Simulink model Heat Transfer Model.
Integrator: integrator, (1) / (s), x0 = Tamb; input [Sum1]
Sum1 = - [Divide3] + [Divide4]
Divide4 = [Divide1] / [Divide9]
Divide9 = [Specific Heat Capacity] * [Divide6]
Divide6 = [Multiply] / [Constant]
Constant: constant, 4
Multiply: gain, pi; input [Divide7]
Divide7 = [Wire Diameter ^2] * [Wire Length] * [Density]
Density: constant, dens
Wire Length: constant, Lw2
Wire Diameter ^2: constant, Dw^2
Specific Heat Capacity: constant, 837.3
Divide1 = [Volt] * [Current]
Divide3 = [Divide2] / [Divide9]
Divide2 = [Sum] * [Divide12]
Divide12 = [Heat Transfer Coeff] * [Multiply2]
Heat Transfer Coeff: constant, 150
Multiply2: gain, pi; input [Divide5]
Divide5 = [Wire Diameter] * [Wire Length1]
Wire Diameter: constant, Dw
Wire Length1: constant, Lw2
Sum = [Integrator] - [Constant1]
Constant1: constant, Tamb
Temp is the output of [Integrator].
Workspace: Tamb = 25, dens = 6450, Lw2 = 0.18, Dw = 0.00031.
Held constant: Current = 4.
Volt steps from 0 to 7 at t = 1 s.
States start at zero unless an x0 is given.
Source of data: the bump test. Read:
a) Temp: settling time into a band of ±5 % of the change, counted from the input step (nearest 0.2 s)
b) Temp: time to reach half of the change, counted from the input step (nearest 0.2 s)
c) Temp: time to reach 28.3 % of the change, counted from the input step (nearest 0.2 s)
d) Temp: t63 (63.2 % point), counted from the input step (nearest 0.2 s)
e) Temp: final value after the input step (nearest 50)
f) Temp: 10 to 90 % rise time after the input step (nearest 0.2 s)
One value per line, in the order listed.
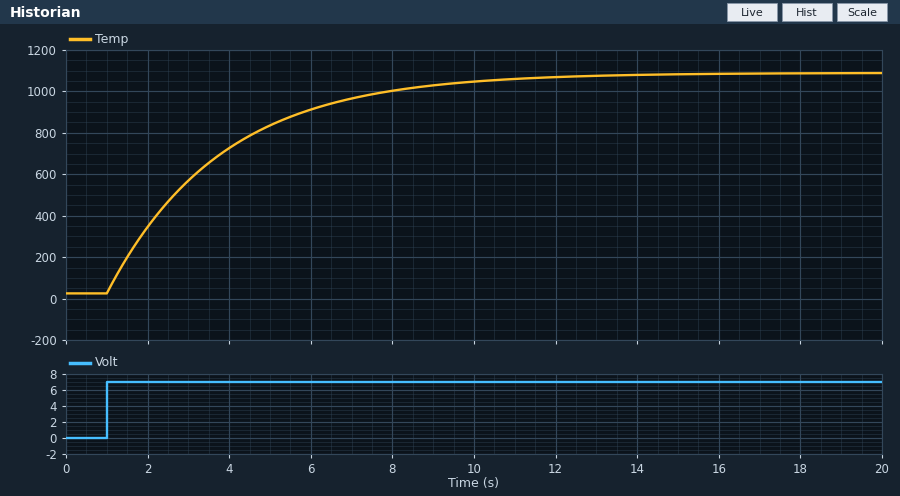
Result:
8.4 s
2.0 s
1.0 s
2.8 s
1100
6.2 s
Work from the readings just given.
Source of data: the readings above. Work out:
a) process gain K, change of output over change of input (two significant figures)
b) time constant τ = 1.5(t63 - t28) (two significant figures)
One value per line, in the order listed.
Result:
160
2.7 s
